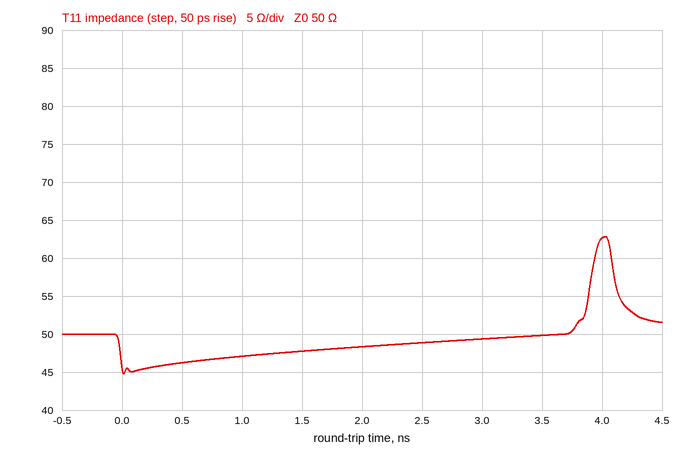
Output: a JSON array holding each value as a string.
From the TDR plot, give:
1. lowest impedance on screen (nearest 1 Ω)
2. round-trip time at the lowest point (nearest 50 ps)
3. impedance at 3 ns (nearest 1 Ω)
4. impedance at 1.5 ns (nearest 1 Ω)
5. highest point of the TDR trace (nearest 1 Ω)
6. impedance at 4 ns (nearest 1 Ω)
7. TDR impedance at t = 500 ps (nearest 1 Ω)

["45 Ω", "0 ps", "49 Ω", "48 Ω", "63 Ω", "63 Ω", "46 Ω"]
